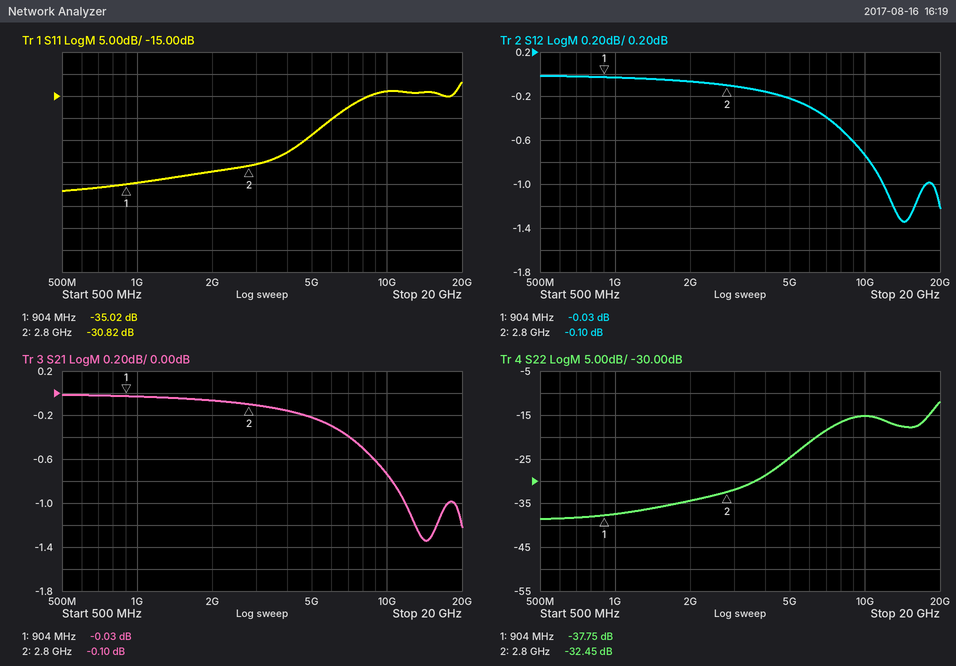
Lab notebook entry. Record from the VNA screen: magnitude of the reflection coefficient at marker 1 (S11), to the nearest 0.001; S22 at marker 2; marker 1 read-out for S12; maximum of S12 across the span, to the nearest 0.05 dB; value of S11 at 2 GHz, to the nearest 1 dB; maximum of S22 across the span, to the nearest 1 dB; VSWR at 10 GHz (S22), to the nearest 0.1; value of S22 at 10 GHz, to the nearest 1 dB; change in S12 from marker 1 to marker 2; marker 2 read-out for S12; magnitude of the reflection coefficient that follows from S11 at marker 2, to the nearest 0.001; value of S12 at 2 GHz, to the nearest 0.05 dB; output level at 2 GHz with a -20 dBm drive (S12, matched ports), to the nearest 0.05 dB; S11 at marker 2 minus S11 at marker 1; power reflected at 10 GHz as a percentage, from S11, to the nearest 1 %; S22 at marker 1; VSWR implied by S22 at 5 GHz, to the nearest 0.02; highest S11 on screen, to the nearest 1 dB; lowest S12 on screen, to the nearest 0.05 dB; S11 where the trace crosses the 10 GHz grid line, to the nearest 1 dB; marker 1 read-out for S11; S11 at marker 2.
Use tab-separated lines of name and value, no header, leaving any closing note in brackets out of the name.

magnitude of the reflection coefficient at marker 1 (S11), to the nearest 0.001	0.018
S22 at marker 2	-32.45 dB
marker 1 read-out for S12	-0.03 dB
maximum of S12 across the span, to the nearest 0.05 dB	0.00 dB
value of S11 at 2 GHz, to the nearest 1 dB	-32 dB
maximum of S22 across the span, to the nearest 1 dB	-12 dB
VSWR at 10 GHz (S22), to the nearest 0.1	1.4
value of S22 at 10 GHz, to the nearest 1 dB	-15 dB
change in S12 from marker 1 to marker 2	-0.07 dB
marker 2 read-out for S12	-0.10 dB
magnitude of the reflection coefficient that follows from S11 at marker 2, to the nearest 0.001	0.029
value of S12 at 2 GHz, to the nearest 0.05 dB	-0.05 dB
output level at 2 GHz with a -20 dBm drive (S12, matched ports), to the nearest 0.05 dB	-20.05 dBm
S11 at marker 2 minus S11 at marker 1	4.20 dB
power reflected at 10 GHz as a percentage, from S11, to the nearest 1 %	4 %
S22 at marker 1	-37.75 dB
VSWR implied by S22 at 5 GHz, to the nearest 0.02	1.12
highest S11 on screen, to the nearest 1 dB	-12 dB
lowest S12 on screen, to the nearest 0.05 dB	-1.35 dB
S11 where the trace crosses the 10 GHz grid line, to the nearest 1 dB	-14 dB
marker 1 read-out for S11	-35.02 dB
S11 at marker 2	-30.82 dB
